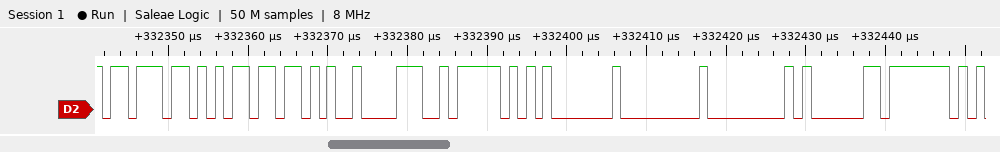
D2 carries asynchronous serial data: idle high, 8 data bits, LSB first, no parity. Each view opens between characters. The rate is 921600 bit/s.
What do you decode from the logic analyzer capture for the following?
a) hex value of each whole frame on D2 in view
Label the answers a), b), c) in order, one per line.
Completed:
a) BB, B5, 2B, 38, 5F, 01, 00, 00, 81, 7F
